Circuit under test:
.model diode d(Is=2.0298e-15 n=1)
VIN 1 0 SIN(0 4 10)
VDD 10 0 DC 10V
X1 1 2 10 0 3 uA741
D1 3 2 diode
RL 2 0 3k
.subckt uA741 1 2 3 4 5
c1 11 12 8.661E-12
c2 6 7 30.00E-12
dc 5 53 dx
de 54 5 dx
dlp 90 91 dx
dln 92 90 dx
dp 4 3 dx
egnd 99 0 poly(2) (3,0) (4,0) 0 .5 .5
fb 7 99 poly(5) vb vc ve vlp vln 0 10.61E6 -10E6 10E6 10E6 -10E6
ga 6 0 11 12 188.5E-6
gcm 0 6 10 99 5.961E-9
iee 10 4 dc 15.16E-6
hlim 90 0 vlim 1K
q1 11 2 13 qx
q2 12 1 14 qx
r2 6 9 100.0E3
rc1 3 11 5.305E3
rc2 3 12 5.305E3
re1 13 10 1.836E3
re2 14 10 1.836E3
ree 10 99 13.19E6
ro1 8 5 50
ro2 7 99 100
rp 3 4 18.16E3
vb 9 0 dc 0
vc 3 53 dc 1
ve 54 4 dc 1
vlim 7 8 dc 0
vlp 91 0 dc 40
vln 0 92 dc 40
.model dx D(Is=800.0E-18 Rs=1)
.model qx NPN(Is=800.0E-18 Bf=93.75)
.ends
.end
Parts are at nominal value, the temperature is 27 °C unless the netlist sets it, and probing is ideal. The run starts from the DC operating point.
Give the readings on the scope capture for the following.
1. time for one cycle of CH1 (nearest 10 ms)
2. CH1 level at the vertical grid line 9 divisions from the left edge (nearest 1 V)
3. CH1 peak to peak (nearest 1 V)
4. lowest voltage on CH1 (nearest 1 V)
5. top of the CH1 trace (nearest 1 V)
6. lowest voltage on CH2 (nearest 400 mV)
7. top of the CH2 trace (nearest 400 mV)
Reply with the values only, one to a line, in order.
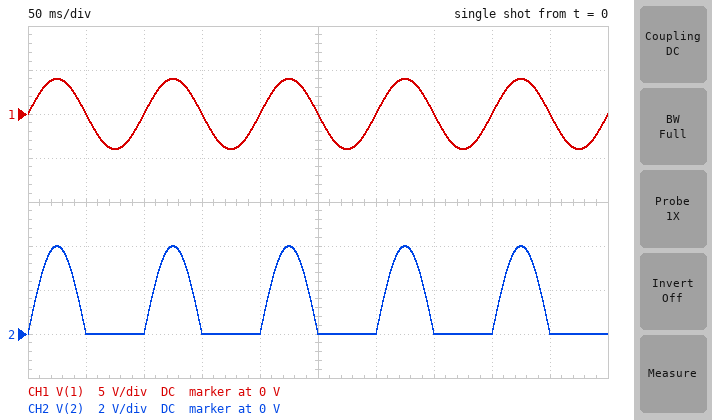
100 ms
0 V
8 V
-4 V
4 V
0 V
4.0 V
